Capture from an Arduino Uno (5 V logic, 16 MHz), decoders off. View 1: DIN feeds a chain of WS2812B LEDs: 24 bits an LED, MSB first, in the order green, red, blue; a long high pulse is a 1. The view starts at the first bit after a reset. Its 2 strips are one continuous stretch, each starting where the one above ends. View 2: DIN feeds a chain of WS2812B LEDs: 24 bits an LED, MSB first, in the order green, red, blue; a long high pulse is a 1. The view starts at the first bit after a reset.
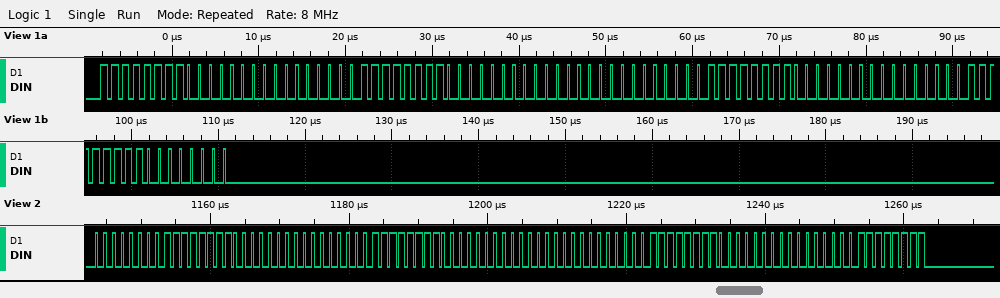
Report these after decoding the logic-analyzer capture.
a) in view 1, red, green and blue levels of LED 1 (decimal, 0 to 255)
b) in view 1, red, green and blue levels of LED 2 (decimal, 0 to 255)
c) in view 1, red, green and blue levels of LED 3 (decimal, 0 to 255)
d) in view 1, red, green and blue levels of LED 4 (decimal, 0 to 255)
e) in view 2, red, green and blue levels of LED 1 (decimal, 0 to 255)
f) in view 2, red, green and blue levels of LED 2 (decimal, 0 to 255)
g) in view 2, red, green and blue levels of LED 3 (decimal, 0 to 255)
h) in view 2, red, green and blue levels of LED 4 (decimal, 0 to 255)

0, 255, 0
0, 255, 0
255, 0, 0
255, 0, 0
255, 0, 0
255, 0, 0
0, 0, 255
0, 0, 255
